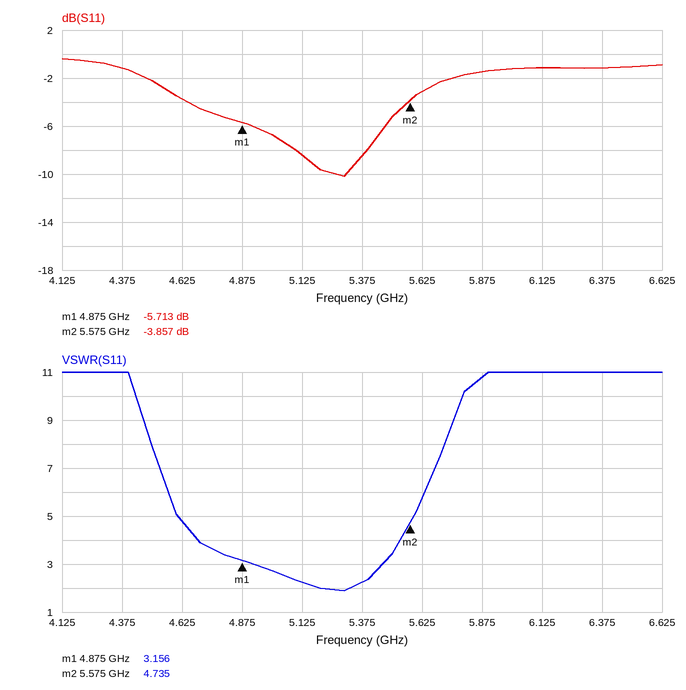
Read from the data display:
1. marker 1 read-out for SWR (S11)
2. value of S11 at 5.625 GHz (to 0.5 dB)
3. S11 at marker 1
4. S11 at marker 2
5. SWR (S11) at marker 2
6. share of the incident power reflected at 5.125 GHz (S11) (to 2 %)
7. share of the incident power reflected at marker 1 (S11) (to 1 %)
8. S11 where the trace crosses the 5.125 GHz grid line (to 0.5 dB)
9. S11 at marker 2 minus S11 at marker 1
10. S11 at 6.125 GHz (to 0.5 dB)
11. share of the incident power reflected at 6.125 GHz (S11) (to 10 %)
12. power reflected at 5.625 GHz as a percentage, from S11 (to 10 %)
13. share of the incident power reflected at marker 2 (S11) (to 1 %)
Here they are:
3.156
-3.0 dB
-5.713 dB
-3.857 dB
4.735
14 %
27 %
-8.5 dB
1.856 dB
-1.0 dB
80 %
50 %
41 %
